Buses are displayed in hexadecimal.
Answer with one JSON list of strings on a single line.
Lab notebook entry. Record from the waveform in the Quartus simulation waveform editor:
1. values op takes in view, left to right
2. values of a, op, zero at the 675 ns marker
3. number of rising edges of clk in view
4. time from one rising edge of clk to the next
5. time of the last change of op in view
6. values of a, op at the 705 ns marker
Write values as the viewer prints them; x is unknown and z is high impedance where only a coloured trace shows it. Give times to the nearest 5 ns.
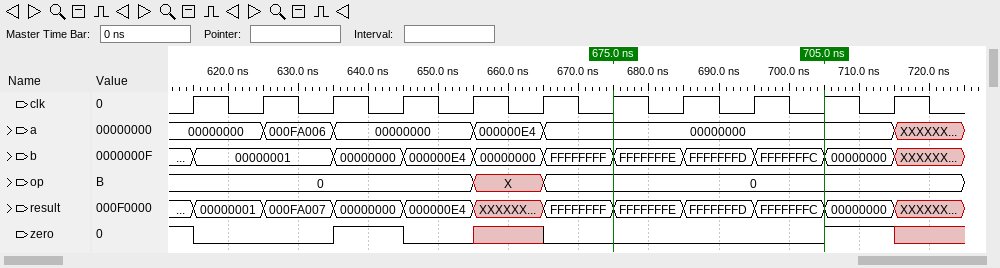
["0, X, 0", "a=00000000, op=0, zero=0", "11", "10 ns", "665 ns", "a=00000000, op=0"]
